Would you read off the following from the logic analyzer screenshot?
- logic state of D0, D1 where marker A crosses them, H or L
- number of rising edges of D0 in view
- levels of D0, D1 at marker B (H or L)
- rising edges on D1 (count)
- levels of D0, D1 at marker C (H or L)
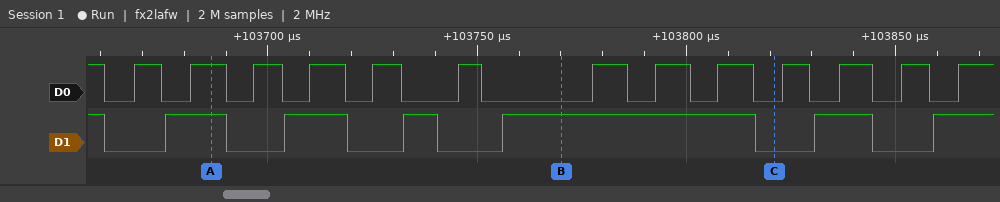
D0=H, D1=H
13
D0=L, D1=H
6
D0=L, D1=L
